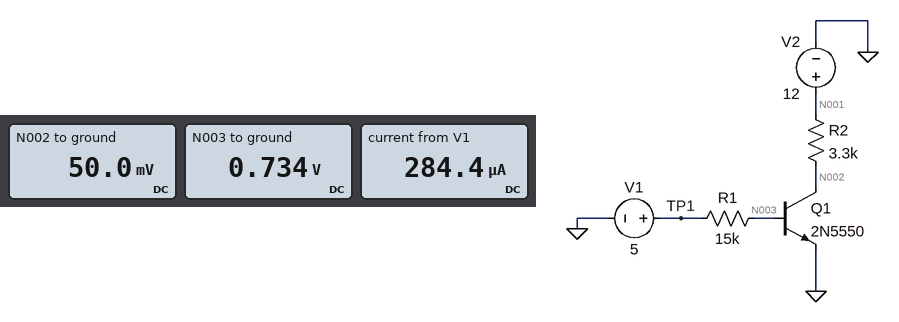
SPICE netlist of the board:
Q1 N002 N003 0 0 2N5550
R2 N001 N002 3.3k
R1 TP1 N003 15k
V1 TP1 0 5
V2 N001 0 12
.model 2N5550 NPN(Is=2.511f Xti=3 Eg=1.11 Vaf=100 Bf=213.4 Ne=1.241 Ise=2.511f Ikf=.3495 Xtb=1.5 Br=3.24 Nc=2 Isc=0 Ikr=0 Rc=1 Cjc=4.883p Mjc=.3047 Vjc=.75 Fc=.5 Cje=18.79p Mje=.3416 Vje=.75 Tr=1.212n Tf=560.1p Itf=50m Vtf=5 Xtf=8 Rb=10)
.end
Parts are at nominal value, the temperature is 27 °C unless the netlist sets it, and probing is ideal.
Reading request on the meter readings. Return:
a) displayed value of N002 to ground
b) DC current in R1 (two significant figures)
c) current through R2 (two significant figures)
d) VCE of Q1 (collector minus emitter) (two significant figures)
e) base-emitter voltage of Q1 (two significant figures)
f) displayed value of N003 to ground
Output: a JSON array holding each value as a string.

["50.0 mV", "280 µA", "3.6 mA", "50 mV", "730 mV", "0.734 V"]
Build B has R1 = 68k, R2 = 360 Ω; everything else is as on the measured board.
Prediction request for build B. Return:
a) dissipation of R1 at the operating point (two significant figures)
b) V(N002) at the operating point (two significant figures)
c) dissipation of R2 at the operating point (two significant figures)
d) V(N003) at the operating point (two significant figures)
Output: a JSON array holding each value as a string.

["270 µW", "9.2 V", "22 mW", "740 mV"]
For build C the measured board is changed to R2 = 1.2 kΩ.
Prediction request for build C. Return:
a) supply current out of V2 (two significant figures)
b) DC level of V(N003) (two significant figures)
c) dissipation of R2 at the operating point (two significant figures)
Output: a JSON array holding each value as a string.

["9.9 mA", "760 mV", "120 mW"]
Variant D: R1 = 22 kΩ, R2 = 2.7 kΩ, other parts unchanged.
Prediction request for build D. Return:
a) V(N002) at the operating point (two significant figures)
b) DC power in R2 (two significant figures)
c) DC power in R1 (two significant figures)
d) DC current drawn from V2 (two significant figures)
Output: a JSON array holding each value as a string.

["66 mV", "53 mW", "830 µW", "4.4 mA"]
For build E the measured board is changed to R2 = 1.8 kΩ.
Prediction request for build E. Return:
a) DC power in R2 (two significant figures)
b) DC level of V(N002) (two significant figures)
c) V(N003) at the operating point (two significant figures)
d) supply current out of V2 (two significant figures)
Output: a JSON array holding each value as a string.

["79 mW", "69 mV", "750 mV", "6.6 mA"]
